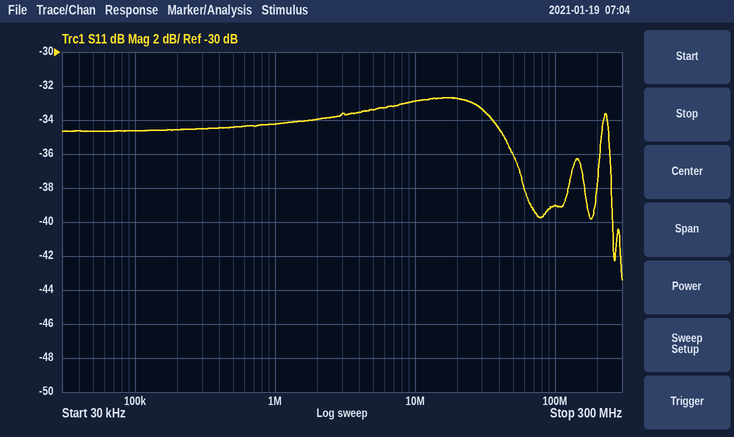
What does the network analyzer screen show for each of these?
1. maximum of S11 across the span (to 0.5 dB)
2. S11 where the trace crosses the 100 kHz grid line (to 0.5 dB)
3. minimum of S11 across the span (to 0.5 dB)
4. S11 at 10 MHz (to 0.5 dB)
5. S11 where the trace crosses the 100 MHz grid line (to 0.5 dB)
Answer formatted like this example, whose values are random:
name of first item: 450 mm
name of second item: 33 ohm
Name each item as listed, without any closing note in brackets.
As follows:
maximum of S11 across the span: -32.5 dB
S11 where the trace crosses the 100 kHz grid line: -34.5 dB
minimum of S11 across the span: -43.5 dB
S11 at 10 MHz: -33.0 dB
S11 where the trace crosses the 100 MHz grid line: -39.0 dB
